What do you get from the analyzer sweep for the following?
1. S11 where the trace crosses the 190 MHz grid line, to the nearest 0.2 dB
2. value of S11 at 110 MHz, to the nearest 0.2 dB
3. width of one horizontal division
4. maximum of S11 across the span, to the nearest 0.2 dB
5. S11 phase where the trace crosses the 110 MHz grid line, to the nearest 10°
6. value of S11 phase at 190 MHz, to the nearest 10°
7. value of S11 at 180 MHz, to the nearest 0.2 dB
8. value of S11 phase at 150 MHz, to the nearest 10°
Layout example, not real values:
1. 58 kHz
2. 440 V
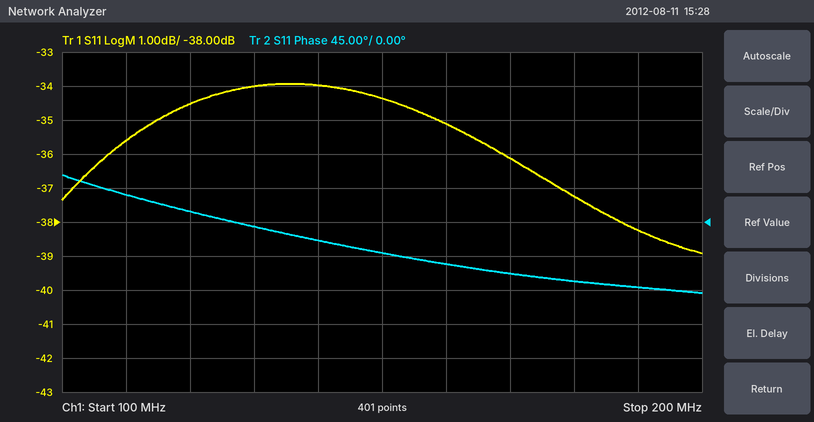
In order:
1. -38.2 dB
2. -35.6 dB
3. 10 MHz
4. -34.0 dB
5. 40°
6. -90°
7. -37.2 dB
8. -40°
